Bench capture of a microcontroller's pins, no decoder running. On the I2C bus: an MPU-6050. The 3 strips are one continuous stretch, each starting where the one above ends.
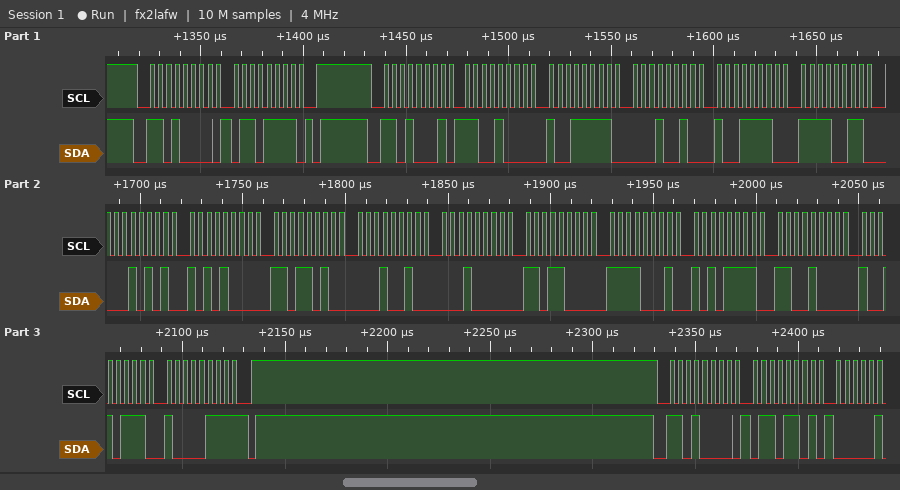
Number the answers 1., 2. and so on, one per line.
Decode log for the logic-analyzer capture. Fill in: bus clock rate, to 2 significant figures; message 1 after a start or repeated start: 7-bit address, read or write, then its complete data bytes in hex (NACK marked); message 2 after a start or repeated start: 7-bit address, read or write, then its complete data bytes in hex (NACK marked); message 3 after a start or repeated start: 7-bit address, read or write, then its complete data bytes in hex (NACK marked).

1. 250 kHz
2. 0x68 write: 6F
3. 0x68 read: C8 9F 12 9E F3 15 A8 DA 12 10 D8 F1 AF C8 97 87 NACK
4. 0x68 write: 6D
